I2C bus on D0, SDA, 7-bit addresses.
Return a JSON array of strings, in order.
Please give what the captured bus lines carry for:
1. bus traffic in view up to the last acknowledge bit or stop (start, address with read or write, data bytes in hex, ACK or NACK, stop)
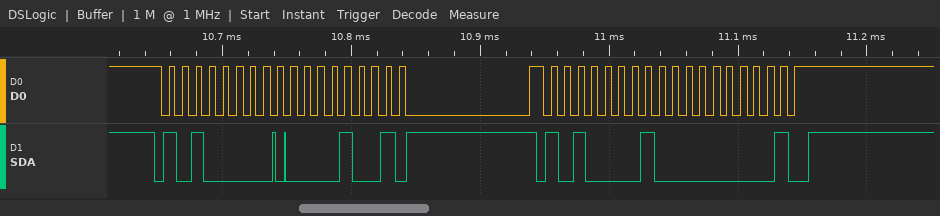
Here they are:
["start, address 50 write ACK, 09 ACK, repeated start, address 50 read ACK, 00 NACK, stop"]
